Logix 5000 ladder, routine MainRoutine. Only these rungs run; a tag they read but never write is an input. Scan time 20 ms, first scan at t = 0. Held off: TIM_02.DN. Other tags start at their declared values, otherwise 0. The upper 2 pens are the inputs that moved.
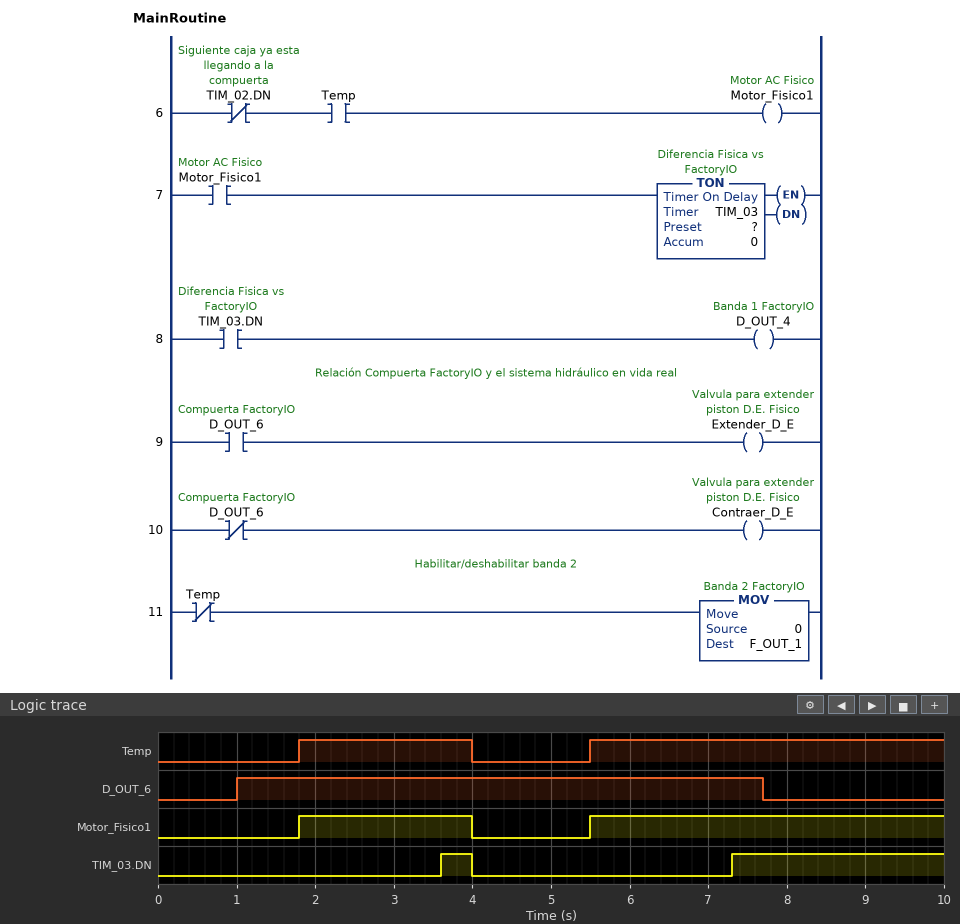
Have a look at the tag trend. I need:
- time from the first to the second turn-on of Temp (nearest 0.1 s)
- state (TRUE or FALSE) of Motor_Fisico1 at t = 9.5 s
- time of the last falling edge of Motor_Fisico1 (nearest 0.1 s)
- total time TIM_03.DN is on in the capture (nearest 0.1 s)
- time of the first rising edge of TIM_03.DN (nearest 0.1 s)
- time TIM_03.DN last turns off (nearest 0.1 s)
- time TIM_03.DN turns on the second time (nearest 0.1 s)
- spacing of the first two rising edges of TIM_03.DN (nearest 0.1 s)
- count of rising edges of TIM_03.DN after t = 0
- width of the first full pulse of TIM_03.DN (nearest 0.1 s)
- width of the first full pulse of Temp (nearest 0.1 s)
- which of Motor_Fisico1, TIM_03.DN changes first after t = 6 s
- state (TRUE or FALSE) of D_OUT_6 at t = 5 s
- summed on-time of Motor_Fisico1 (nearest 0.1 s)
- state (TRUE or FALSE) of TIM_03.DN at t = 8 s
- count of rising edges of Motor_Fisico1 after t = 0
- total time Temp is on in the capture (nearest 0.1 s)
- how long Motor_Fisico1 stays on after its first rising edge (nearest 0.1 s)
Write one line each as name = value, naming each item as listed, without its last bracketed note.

time from the first to the second turn-on of Temp = 3.7 s
state (TRUE or FALSE) of Motor_Fisico1 at t = 9.5 s = TRUE
time of the last falling edge of Motor_Fisico1 = 4.0 s
total time TIM_03.DN is on in the capture = 3.1 s
time of the first rising edge of TIM_03.DN = 3.6 s
time TIM_03.DN last turns off = 4.0 s
time TIM_03.DN turns on the second time = 7.3 s
spacing of the first two rising edges of TIM_03.DN = 3.7 s
count of rising edges of TIM_03.DN after t = 0 = 2
width of the first full pulse of TIM_03.DN = 0.4 s
width of the first full pulse of Temp = 2.2 s
which of Motor_Fisico1, TIM_03.DN changes first after t = 6 s = TIM_03.DN
state (TRUE or FALSE) of D_OUT_6 at t = 5 s = TRUE
summed on-time of Motor_Fisico1 = 6.7 s
state (TRUE or FALSE) of TIM_03.DN at t = 8 s = TRUE
count of rising edges of Motor_Fisico1 after t = 0 = 2
total time Temp is on in the capture = 6.7 s
how long Motor_Fisico1 stays on after its first rising edge = 2.2 s
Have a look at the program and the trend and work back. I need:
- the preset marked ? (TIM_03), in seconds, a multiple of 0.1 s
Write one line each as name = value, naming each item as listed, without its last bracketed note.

the preset marked ? (TIM_03), in seconds, a multiple of 0.1 s = 1.8 s
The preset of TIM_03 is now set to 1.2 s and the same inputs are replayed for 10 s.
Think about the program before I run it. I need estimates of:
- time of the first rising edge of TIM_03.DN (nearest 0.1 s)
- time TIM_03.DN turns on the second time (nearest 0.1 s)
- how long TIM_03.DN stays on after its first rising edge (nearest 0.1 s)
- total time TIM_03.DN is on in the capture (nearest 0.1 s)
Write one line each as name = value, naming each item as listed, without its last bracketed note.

time of the first rising edge of TIM_03.DN = 3.0 s
time TIM_03.DN turns on the second time = 6.7 s
how long TIM_03.DN stays on after its first rising edge = 1.0 s
total time TIM_03.DN is on in the capture = 4.3 s
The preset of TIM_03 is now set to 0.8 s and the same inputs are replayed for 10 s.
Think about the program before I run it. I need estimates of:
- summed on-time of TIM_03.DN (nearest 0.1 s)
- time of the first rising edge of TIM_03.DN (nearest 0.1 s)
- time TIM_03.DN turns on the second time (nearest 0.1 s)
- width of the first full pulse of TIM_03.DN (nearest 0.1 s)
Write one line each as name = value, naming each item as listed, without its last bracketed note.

summed on-time of TIM_03.DN = 5.1 s
time of the first rising edge of TIM_03.DN = 2.6 s
time TIM_03.DN turns on the second time = 6.3 s
width of the first full pulse of TIM_03.DN = 1.4 s
